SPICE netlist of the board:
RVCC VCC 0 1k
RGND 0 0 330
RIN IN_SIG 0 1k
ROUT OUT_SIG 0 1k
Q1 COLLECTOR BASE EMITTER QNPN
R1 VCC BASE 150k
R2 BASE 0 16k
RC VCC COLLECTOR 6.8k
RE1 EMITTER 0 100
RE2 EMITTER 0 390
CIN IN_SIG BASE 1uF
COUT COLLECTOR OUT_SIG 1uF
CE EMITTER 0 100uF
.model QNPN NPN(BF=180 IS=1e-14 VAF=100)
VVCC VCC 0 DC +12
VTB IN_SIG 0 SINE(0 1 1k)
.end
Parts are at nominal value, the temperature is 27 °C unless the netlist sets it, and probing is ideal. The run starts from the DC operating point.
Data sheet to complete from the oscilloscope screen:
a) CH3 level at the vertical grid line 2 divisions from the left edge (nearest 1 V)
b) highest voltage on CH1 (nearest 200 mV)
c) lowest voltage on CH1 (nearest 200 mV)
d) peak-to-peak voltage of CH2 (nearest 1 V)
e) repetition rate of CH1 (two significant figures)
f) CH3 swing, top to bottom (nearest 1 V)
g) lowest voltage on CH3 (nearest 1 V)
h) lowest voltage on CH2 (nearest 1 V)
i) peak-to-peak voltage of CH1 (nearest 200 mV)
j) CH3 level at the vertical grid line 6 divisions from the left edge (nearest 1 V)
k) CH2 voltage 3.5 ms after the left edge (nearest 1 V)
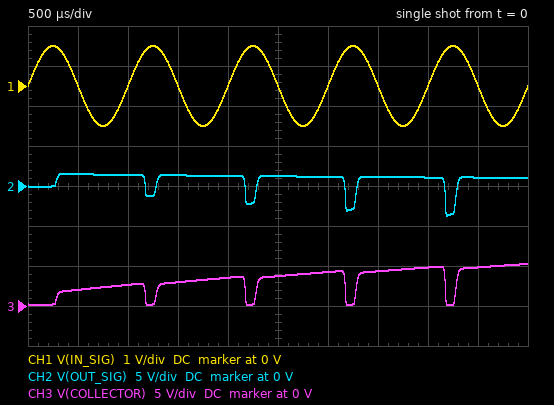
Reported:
3 V
1.0 V
-1.0 V
5 V
1.0 kHz
5 V
0 V
-4 V
2.0 V
4 V
1 V
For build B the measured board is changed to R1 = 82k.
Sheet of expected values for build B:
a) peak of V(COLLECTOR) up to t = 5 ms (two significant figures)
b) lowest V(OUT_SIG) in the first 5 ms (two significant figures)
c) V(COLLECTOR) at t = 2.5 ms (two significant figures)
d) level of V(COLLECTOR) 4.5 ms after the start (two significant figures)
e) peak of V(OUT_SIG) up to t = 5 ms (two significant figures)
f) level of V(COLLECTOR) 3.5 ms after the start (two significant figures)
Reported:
5.1 V
-3.6 V
3.6 V
4.6 V
1.5 V
4.2 V
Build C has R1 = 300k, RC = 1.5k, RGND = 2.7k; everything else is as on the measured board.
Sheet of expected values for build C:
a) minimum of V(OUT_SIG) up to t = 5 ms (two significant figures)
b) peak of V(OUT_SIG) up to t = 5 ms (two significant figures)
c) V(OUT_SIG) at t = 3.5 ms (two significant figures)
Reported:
-12 V
1.1 V
1.0 V
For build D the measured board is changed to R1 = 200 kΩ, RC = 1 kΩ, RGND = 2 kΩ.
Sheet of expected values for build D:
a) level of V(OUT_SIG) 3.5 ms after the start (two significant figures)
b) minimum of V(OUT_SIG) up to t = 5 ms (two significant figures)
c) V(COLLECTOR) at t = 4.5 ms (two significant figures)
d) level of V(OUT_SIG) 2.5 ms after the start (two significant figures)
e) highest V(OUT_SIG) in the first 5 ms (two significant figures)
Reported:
1.3 V
-10 V
11 V
1.4 V
1.9 V
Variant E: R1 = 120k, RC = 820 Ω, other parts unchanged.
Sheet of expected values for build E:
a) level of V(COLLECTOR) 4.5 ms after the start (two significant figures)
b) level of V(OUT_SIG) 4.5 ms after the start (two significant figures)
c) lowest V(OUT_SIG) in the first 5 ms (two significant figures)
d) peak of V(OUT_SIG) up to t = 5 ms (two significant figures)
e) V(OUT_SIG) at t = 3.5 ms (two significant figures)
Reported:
11 V
1.5 V
-9.5 V
3.0 V
1.6 V
